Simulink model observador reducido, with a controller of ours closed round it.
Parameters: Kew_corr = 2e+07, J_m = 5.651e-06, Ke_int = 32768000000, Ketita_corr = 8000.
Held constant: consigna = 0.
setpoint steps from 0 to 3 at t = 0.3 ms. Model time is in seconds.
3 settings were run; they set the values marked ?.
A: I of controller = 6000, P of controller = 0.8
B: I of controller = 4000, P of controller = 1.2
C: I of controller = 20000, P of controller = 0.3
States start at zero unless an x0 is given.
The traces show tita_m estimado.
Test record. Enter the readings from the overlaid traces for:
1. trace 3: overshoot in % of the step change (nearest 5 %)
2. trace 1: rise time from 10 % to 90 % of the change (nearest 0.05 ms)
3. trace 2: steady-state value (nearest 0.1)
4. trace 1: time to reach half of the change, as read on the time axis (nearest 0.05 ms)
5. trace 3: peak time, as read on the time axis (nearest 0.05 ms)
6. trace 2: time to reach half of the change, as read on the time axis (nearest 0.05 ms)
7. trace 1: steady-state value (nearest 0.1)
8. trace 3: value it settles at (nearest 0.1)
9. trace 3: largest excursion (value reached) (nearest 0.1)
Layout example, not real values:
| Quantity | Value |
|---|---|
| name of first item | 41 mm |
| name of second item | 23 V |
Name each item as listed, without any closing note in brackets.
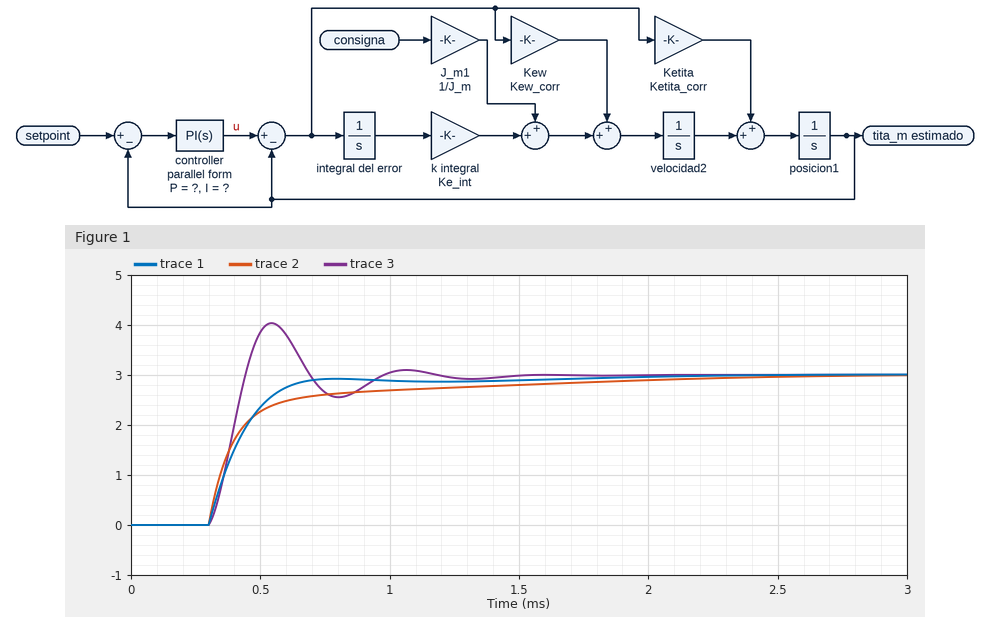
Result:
| Quantity | Value |
|---|---|
| trace 3: overshoot in % of the step change | 35 % |
| trace 1: rise time from 10 % to 90 % of the change | 0.25 ms |
| trace 2: steady-state value | 3.0 |
| trace 1: time to reach half of the change, as read on the time axis | 0.40 ms |
| trace 3: peak time, as read on the time axis | 0.55 ms |
| trace 2: time to reach half of the change, as read on the time axis | 0.40 ms |
| trace 1: steady-state value | 3.0 |
| trace 3: value it settles at | 3.0 |
| trace 3: largest excursion (value reached) | 4.0 |
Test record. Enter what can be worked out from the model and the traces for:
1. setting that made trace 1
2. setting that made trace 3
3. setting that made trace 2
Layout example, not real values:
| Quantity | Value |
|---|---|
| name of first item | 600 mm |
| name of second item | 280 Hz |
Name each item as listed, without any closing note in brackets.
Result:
| Quantity | Value |
|---|---|
| setting that made trace 1 | A |
| setting that made trace 3 | C |
| setting that made trace 2 | B |
